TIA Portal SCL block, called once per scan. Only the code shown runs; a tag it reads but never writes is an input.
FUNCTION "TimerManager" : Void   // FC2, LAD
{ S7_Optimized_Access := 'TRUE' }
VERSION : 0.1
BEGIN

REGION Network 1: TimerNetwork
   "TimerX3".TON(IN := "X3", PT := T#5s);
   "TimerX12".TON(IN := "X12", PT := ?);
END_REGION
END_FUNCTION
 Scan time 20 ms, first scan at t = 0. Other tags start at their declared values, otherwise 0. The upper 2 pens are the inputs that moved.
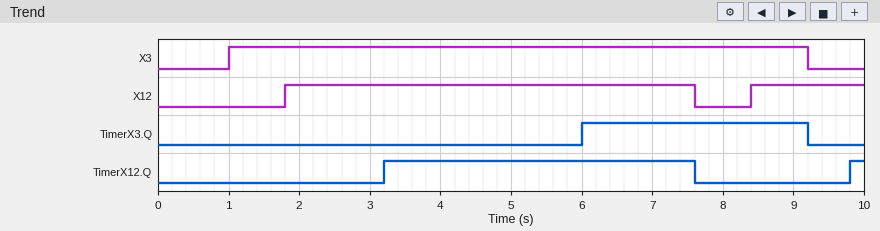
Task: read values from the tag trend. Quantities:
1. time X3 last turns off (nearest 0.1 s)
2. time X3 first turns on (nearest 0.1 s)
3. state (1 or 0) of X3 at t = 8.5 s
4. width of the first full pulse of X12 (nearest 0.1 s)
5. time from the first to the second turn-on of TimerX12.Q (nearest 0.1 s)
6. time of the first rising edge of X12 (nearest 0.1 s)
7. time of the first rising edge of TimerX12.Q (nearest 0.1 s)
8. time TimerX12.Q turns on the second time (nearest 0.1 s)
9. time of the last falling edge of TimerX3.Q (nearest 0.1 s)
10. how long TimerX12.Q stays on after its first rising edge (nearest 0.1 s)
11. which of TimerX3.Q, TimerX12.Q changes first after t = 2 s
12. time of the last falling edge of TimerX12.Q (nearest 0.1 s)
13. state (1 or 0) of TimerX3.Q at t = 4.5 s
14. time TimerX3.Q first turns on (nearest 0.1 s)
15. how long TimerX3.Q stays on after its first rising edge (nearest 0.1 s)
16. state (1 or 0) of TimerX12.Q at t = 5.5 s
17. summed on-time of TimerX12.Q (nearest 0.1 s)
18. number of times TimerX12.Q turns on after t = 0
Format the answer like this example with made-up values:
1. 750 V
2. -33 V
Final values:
1. 9.2 s
2. 1.0 s
3. 1
4. 5.8 s
5. 6.6 s
6. 1.8 s
7. 3.2 s
8. 9.8 s
9. 9.2 s
10. 4.4 s
11. TimerX12.Q
12. 7.6 s
13. 0
14. 6.0 s
15. 3.2 s
16. 1
17. 4.6 s
18. 2
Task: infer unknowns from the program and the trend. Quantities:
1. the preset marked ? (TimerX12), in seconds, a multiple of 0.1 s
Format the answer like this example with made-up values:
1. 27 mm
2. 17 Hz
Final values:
1. 1.4 s
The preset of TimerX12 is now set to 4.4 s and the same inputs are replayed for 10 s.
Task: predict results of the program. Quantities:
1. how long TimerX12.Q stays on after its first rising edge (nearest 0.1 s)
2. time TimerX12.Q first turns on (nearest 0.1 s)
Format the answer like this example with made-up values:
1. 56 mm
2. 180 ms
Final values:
1. 1.4 s
2. 6.2 s
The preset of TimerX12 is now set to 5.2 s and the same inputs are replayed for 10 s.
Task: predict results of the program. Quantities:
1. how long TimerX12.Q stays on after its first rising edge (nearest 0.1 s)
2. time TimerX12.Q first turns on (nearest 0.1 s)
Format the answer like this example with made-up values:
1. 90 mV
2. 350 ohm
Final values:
1. 0.6 s
2. 7.0 s
